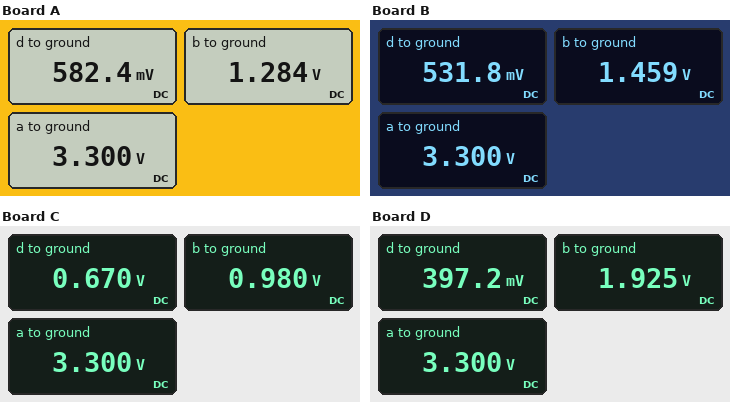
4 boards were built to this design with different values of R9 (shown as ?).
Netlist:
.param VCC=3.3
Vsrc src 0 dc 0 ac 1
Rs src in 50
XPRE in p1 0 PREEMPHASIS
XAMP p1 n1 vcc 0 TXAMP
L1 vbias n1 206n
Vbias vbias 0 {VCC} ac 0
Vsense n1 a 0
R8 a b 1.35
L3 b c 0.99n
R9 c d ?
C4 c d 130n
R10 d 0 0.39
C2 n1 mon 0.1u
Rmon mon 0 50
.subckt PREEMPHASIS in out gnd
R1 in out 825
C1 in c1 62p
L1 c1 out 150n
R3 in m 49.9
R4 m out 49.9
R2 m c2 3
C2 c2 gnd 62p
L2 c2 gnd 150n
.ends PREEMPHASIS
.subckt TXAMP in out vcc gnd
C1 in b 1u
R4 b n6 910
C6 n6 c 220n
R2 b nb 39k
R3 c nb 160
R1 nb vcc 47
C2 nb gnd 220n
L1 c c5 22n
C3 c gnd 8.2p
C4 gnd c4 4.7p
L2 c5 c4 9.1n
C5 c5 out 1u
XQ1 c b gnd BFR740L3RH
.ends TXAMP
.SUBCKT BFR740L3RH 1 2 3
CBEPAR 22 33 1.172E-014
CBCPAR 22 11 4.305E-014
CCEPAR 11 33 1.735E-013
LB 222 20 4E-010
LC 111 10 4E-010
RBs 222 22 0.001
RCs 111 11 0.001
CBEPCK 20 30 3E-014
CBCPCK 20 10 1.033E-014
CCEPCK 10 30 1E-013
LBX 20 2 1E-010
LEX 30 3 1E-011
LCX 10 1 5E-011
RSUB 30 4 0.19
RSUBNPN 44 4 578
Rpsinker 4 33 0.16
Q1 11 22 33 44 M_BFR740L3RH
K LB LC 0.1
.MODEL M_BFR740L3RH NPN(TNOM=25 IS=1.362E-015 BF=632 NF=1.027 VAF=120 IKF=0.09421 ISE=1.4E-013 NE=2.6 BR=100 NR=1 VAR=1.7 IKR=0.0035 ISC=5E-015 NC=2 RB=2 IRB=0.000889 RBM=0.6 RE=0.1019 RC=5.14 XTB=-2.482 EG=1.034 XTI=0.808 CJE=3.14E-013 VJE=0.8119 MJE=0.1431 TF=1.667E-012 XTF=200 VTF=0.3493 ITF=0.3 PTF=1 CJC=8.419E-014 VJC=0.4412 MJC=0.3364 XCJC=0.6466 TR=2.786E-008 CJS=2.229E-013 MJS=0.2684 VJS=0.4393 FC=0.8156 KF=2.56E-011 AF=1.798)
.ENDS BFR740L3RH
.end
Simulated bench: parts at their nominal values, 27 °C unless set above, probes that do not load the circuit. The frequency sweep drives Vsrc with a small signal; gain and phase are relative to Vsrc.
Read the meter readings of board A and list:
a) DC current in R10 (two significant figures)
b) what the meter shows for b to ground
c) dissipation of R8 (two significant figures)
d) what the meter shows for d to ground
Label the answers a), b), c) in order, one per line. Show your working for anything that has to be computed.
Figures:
a) (582.4 mV) / 390 mΩ = 1.5 A
b) 1.284 V
c) (3.3 V - 1.284 V)^2 / 1.35 Ω = 3.0 W
d) 582.4 mV
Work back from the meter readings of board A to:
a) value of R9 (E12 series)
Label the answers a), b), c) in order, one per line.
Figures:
a) 0.47 Ω
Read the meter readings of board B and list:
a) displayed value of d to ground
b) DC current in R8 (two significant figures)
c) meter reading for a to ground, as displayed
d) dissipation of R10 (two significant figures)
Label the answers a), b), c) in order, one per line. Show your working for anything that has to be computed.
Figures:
a) 531.8 mV
b) (3.3 V - 1.459 V) / 1.35 Ω = 1.4 A
c) 3.300 V
d) (531.8 mV)^2 / 390 mΩ = 730 mW
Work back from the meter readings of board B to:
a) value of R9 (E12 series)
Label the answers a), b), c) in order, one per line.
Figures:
a) 0.68 Ω
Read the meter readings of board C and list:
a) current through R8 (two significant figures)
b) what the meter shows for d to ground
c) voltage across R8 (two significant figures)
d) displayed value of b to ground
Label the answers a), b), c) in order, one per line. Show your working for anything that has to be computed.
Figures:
a) (3.3 V - 980 mV) / 1.35 Ω = 1.7 A
b) 0.670 V
c) 3.3 V - 980 mV = 2.3 V
d) 0.980 V
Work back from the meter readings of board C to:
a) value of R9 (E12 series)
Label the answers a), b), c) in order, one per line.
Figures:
a) 0.18 Ω
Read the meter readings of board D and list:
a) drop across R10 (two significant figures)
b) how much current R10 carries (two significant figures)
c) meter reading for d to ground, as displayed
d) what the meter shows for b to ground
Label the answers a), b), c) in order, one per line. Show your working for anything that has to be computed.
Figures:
a) 397.2 mV = 400 mV
b) (397.2 mV) / 390 mΩ = 1.0 A
c) 397.2 mV
d) 1.925 V
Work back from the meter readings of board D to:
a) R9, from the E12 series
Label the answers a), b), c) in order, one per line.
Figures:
a) 1.5 Ω
